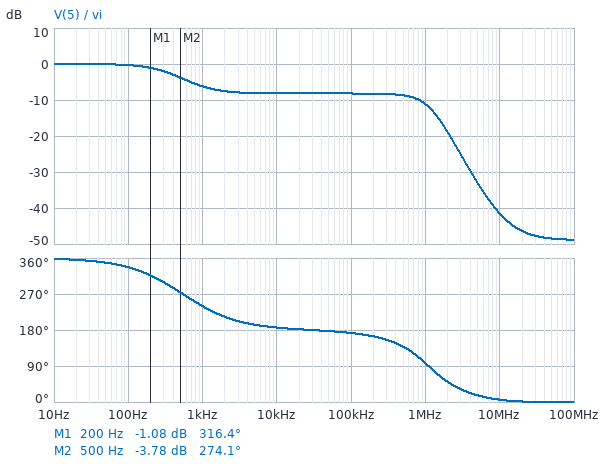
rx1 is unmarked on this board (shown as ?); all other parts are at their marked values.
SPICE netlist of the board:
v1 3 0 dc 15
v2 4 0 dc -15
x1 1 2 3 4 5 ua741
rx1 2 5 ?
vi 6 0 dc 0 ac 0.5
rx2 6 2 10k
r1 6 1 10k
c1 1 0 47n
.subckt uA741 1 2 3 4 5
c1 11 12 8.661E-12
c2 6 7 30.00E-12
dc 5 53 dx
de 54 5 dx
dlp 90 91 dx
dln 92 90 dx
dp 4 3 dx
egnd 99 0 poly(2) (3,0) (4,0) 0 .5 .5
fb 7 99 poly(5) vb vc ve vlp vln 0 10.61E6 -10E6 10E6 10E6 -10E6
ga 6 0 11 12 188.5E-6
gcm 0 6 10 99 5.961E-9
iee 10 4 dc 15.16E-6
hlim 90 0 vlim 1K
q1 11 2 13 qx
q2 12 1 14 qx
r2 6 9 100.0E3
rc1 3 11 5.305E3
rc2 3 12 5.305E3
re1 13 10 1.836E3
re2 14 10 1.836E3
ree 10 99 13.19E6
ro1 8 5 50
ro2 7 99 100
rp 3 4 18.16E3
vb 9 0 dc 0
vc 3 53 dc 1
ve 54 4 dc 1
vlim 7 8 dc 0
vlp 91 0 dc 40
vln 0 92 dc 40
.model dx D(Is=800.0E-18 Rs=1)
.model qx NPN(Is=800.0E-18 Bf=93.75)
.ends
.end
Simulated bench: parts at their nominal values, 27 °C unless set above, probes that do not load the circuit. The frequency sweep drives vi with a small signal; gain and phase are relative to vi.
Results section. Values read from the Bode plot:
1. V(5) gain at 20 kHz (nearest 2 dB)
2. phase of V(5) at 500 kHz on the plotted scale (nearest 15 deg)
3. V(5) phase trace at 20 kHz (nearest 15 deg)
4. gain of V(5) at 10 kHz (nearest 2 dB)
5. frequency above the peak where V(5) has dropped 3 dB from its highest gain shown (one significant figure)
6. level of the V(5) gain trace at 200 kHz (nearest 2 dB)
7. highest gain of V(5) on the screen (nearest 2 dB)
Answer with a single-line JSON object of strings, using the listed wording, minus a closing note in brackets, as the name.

{"V(5) gain at 20 kHz": "-8 dB", "phase of V(5) at 500 kHz on the plotted scale": "135 deg", "V(5) phase trace at 20 kHz": "180 deg", "gain of V(5) at 10 kHz": "-8 dB", "frequency above the peak where V(5) has dropped 3 dB from its highest gain shown": "400 Hz", "level of the V(5) gain trace at 200 kHz": "-8 dB", "highest gain of V(5) on the screen": "0 dB"}
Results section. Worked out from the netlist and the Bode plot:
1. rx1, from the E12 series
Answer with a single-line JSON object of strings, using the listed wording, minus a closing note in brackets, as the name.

{"rx1, from the E12 series": "3.9 kΩ"}
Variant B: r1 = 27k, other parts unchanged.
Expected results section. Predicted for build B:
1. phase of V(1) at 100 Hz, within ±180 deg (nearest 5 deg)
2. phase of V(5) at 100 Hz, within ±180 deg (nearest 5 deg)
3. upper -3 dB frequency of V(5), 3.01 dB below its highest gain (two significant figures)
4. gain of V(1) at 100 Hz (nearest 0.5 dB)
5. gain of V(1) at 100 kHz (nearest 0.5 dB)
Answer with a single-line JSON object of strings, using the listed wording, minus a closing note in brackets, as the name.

{"phase of V(1) at 100 Hz, within ±180 deg": "-40 deg", "phase of V(5) at 100 Hz, within ±180 deg": "-55 deg", "upper -3 dB frequency of V(5), 3.01 dB below its highest gain": "150 Hz", "gain of V(1) at 100 Hz": "-2.0 dB", "gain of V(1) at 100 kHz": "-58.0 dB"}
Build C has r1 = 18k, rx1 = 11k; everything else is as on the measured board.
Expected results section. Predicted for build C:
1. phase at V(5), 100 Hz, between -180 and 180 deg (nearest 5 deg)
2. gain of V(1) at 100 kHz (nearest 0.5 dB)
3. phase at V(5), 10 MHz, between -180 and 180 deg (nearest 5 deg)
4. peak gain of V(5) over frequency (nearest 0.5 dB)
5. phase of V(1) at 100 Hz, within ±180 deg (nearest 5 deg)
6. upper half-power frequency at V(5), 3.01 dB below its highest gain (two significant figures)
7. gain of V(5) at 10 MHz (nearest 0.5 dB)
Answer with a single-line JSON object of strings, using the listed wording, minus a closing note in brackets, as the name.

{"phase at V(5), 100 Hz, between -180 and 180 deg": "-60 deg", "gain of V(1) at 100 kHz": "-54.5 dB", "phase at V(5), 10 MHz, between -180 and 180 deg": "10 deg", "peak gain of V(5) over frequency": "1.0 dB", "phase of V(1) at 100 Hz, within ±180 deg": "-30 deg", "upper half-power frequency at V(5), 3.01 dB below its highest gain": "620 kHz", "gain of V(5) at 10 MHz": "-39.0 dB"}
